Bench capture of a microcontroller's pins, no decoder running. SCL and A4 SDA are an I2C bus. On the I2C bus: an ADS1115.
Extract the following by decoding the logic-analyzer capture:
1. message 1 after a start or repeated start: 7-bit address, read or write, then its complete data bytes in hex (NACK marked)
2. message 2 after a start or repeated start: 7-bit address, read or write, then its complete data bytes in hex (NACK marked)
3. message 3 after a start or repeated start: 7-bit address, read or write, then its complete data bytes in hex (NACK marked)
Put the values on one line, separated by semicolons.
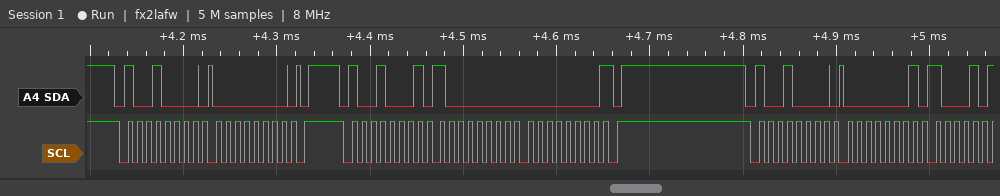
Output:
0x48 write: 00; 0x48 read: 80 00 NACK; 0x48 write: 01
